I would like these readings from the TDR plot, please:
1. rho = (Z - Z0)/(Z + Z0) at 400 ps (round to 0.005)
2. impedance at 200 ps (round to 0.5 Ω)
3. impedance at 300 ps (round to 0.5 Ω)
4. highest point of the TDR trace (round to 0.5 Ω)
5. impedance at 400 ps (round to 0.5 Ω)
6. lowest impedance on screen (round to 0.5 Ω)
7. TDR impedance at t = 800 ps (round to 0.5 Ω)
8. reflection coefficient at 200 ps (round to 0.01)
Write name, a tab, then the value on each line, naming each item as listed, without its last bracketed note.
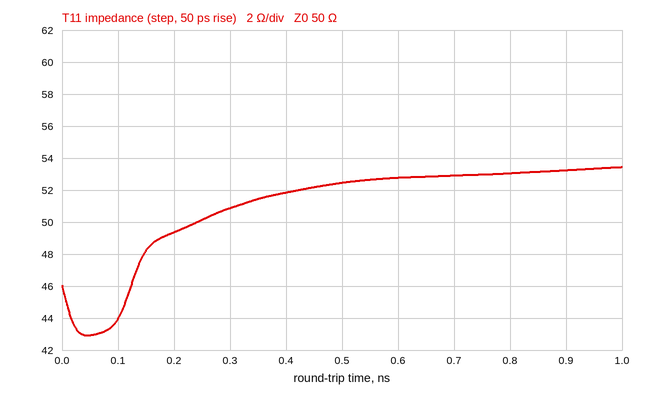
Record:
rho = (Z - Z0)/(Z + Z0) at 400 ps	+0.020
impedance at 200 ps	49.5 Ω
impedance at 300 ps	51.0 Ω
highest point of the TDR trace	53.5 Ω
impedance at 400 ps	52.0 Ω
lowest impedance on screen	43.0 Ω
TDR impedance at t = 800 ps	53.0 Ω
reflection coefficient at 200 ps	-0.01
